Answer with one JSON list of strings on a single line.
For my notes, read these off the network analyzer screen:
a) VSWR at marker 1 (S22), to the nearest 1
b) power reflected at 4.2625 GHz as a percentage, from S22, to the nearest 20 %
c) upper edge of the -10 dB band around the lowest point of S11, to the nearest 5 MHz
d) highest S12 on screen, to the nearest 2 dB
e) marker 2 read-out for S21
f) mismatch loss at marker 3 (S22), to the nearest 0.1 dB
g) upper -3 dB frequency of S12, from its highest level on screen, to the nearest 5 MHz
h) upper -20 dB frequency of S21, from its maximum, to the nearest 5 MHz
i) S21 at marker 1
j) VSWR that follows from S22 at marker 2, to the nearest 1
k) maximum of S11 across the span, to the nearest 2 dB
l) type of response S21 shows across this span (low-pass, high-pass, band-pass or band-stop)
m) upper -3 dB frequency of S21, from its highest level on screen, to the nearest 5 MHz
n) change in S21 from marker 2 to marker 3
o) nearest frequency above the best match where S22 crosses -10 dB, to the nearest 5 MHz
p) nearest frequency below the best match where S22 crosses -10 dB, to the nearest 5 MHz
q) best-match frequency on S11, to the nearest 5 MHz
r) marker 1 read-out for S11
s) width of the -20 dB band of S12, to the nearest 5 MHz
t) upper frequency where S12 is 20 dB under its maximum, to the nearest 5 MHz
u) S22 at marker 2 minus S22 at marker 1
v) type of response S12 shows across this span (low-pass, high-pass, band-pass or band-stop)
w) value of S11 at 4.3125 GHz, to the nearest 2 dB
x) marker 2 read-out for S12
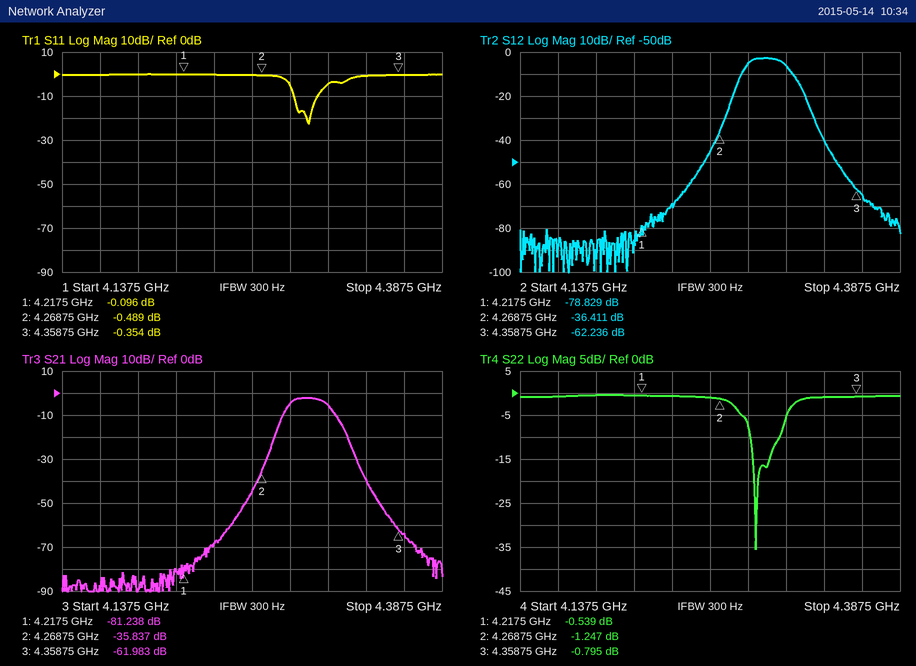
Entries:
["32", "80 %", "4.305 GHz", "-2 dB", "-35.837 dB", "7.8 dB", "4.310 GHz", "4.325 GHz", "-81.238 dB", "14", "0 dB", "band-pass", "4.310 GHz", "-26.146 dB", "4.310 GHz", "4.290 GHz", "4.300 GHz", "-0.096 dB", "50 MHz", "4.325 GHz", "-0.708 dB", "band-pass", "-4 dB", "-36.411 dB"]
